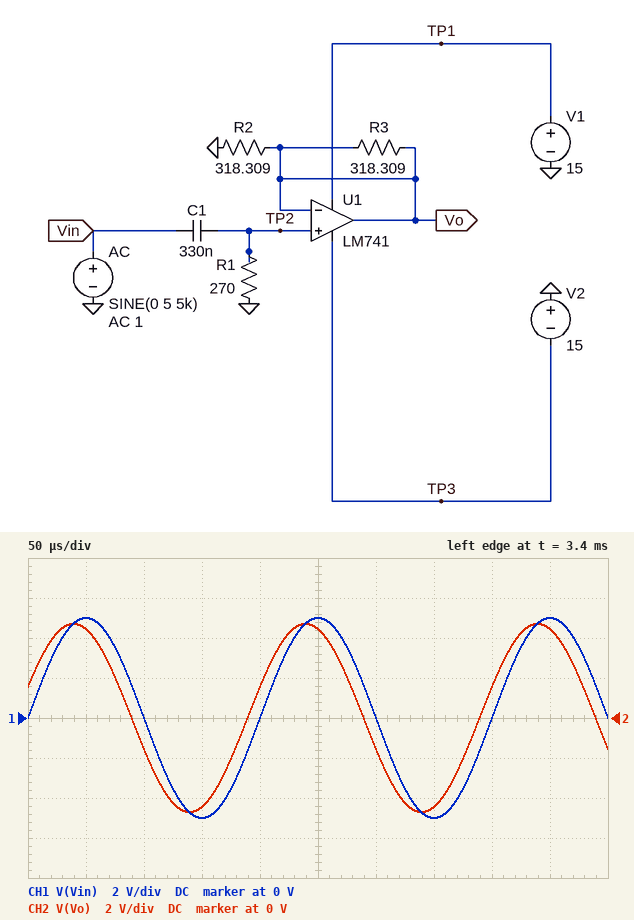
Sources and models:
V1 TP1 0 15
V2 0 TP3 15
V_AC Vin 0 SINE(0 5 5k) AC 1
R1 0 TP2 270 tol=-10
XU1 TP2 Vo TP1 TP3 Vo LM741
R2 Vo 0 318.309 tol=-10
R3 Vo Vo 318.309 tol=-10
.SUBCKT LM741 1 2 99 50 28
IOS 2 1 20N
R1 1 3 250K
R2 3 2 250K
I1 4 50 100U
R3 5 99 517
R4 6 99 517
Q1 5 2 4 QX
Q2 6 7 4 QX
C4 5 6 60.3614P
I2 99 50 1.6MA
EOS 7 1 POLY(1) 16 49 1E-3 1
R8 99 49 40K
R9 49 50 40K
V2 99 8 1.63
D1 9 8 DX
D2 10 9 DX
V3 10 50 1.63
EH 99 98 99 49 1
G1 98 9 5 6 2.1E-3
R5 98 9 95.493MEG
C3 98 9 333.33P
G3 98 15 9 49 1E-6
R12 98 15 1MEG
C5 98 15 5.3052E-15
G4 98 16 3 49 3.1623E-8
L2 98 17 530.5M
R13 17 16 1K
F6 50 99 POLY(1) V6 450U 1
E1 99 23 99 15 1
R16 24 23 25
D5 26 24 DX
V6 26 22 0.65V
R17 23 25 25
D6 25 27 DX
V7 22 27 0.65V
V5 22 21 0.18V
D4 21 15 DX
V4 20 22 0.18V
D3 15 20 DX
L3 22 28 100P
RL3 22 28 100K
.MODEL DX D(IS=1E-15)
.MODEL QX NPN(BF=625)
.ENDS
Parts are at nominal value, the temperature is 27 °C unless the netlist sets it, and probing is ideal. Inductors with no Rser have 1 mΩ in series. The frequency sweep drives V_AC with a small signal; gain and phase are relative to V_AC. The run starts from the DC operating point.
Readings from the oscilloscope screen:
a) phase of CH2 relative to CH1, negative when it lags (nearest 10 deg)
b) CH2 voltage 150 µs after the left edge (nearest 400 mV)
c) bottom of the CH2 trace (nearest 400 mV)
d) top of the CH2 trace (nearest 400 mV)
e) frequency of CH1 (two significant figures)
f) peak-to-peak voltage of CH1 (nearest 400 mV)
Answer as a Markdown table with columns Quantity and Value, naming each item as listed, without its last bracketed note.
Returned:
| Quantity | Value |
|---|---|
| phase of CH2 relative to CH1, negative when it lags | 20 deg |
| CH2 voltage 150 µs after the left edge | -4.4 V |
| bottom of the CH2 trace | -4.8 V |
| top of the CH2 trace | 4.8 V |
| frequency of CH1 | 5.0 kHz |
| peak-to-peak voltage of CH1 | 10.0 V |
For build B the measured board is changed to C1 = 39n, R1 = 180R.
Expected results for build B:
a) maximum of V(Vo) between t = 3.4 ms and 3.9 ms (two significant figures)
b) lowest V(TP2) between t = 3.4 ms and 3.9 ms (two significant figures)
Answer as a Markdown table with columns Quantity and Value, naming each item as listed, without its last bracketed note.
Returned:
| Quantity | Value |
|---|---|
| maximum of V(Vo) between t = 3.4 ms and 3.9 ms | 1.1 V |
| lowest V(TP2) between t = 3.4 ms and 3.9 ms | -1.1 V |
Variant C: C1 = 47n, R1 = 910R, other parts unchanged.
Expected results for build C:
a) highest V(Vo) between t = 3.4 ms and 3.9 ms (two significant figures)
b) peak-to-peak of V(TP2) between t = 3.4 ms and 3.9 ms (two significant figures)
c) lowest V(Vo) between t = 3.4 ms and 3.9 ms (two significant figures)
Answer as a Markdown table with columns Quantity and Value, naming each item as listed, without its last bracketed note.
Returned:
| Quantity | Value |
|---|---|
| highest V(Vo) between t = 3.4 ms and 3.9 ms | 4.0 V |
| peak-to-peak of V(TP2) between t = 3.4 ms and 3.9 ms | 8.0 V |
| lowest V(Vo) between t = 3.4 ms and 3.9 ms | -4.0 V |
